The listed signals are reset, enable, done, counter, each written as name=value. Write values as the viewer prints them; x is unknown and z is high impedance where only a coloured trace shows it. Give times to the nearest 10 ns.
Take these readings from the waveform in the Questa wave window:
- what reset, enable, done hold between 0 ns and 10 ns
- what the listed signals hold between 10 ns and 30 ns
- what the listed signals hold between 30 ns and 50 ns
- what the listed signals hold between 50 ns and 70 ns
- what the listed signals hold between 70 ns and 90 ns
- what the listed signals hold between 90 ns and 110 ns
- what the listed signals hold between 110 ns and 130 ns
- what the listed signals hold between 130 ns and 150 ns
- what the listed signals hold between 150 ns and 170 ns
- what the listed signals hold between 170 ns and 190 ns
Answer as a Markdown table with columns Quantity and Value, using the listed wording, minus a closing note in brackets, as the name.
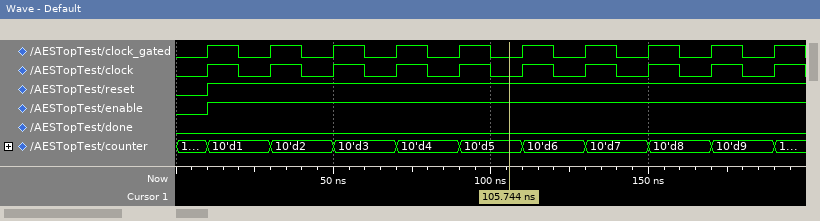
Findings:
| Quantity | Value |
|---|---|
| what reset, enable, done hold between 0 ns and 10 ns | reset=0, enable=0, done=0 |
| what the listed signals hold between 10 ns and 30 ns | reset=1, enable=1, done=0, counter=10'd1 |
| what the listed signals hold between 30 ns and 50 ns | reset=1, enable=1, done=0, counter=10'd2 |
| what the listed signals hold between 50 ns and 70 ns | reset=1, enable=1, done=0, counter=10'd3 |
| what the listed signals hold between 70 ns and 90 ns | reset=1, enable=1, done=0, counter=10'd4 |
| what the listed signals hold between 90 ns and 110 ns | reset=1, enable=1, done=0, counter=10'd5 |
| what the listed signals hold between 110 ns and 130 ns | reset=1, enable=1, done=0, counter=10'd6 |
| what the listed signals hold between 130 ns and 150 ns | reset=1, enable=1, done=0, counter=10'd7 |
| what the listed signals hold between 150 ns and 170 ns | reset=1, enable=1, done=0, counter=10'd8 |
| what the listed signals hold between 170 ns and 190 ns | reset=1, enable=1, done=0, counter=10'd9 |
